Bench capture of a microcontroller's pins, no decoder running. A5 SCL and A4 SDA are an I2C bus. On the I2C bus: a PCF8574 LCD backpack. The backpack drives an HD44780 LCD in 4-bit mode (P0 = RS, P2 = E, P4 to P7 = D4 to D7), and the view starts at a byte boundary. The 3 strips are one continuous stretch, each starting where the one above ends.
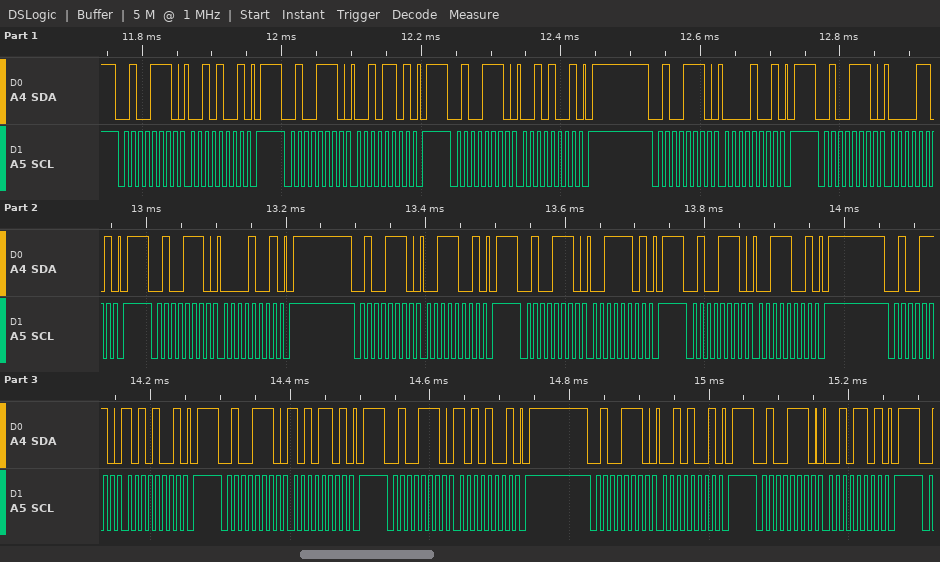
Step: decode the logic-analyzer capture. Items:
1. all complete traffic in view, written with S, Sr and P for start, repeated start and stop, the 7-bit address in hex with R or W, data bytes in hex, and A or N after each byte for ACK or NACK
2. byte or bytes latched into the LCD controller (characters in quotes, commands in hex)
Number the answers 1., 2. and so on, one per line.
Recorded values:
1. S 27W A 29 A P S 27W A 2D A P S 27W A 29 A P S 27W A 09 A P S 27W A 0D A P S 27W A 09 A P S 27W A 39 A P S 27W A 3D A P S 27W A 39 A P S 27W A A9 A P S 27W A AD A P S 27W A A9 A P S 27W A 29 A P S 27W A 2D A P
2. ' ' ':'
